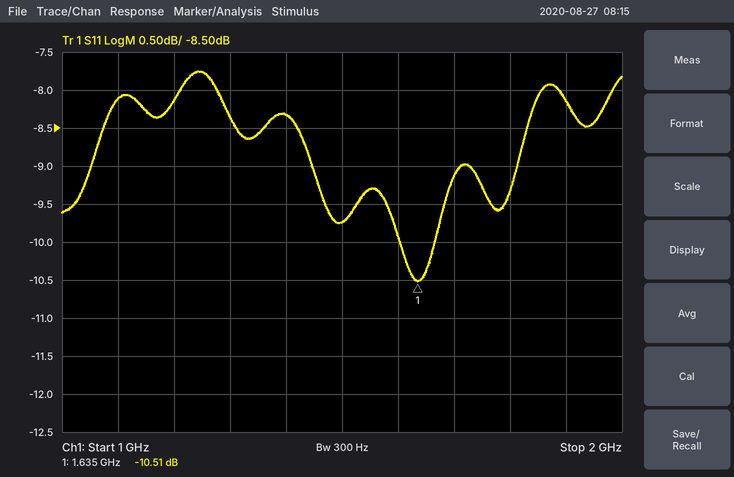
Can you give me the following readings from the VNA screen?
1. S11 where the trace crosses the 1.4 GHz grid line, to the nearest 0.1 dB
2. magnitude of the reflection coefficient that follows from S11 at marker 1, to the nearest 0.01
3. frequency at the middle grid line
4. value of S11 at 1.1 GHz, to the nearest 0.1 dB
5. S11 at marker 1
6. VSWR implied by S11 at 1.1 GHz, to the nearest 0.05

-8.3 dB
0.30
1.5 GHz
-8.1 dB
-10.51 dB
2.30
